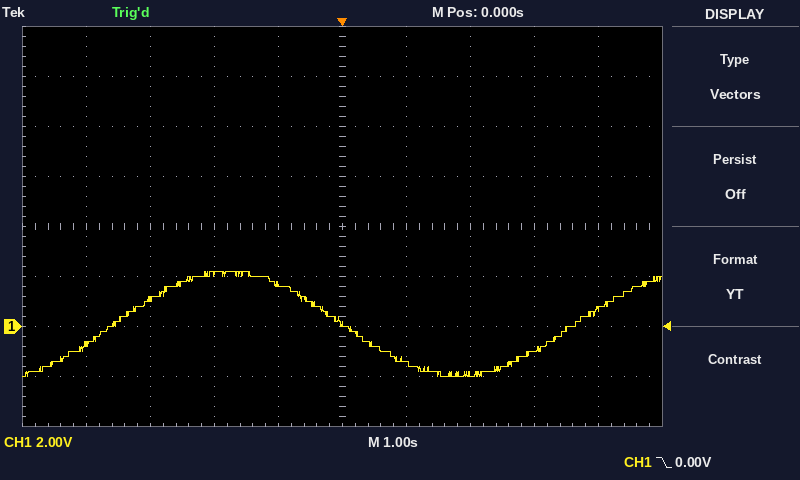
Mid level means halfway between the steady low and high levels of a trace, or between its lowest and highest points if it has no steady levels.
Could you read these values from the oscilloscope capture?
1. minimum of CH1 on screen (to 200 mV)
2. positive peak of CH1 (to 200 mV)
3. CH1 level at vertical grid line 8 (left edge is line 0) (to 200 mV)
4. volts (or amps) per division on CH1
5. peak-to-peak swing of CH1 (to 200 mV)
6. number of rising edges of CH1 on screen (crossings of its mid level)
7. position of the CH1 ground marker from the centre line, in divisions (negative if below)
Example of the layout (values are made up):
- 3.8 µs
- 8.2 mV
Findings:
- -2.0 V
- 2.2 V
- -1.0 V
- 2 V
- 4.2 V
- 2
- -2.0 div
